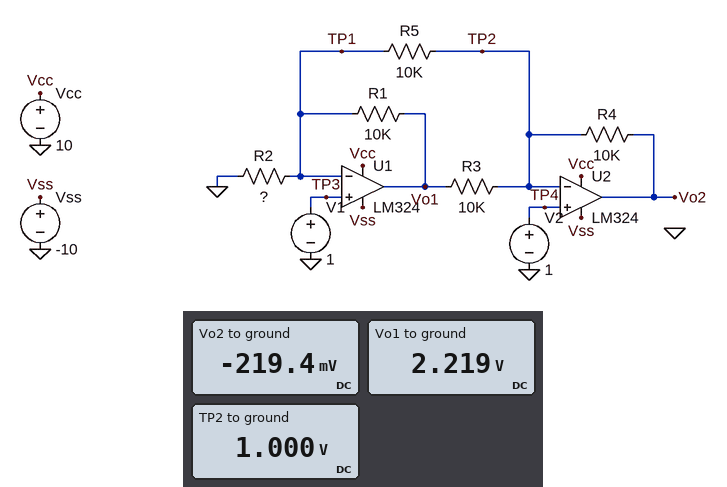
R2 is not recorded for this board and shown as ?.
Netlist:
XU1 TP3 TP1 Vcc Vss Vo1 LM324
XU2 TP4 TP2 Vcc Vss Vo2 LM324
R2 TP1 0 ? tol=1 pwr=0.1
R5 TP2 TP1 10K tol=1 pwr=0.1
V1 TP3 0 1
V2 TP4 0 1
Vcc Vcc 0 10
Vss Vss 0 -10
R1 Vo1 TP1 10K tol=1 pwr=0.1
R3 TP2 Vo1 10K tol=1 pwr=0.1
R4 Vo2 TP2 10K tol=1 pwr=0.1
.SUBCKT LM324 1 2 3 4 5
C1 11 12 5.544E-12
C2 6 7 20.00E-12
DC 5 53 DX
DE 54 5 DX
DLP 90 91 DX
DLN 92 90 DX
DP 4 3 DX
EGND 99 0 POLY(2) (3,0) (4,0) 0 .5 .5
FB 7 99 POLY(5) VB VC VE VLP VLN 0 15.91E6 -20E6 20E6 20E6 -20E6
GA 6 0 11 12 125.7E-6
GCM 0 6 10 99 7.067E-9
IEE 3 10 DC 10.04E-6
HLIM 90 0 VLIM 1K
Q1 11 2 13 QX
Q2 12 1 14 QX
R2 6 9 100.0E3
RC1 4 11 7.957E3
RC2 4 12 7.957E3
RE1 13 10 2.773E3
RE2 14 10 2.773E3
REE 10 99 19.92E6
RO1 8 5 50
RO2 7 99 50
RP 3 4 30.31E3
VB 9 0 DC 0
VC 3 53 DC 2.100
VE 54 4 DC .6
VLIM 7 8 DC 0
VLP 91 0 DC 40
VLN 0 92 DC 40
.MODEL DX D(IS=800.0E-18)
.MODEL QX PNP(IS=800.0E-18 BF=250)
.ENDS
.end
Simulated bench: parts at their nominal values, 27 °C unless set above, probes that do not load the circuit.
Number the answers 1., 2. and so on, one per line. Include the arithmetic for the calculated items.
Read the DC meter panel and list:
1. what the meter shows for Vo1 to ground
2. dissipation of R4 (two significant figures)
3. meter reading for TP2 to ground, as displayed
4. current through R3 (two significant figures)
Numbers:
1. 2.219 V
2. (1 V - (-219.4 mV))^2 / 10 kΩ = 150 µW
3. 1.000 V
4. (2.219 V - 1 V) / 10 kΩ = 120 µA
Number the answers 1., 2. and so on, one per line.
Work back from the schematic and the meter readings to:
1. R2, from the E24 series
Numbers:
1. 8.2 kΩ
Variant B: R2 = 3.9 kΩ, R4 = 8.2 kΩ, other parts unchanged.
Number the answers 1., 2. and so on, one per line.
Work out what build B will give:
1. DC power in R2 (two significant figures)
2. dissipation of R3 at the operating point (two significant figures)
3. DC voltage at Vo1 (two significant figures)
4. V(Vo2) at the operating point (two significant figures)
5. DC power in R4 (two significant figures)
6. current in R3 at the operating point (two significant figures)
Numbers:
1. 260 µW
2. 660 µW
3. 3.6 V
4. -1.1 V
5. 540 µW
6. 260 µA
